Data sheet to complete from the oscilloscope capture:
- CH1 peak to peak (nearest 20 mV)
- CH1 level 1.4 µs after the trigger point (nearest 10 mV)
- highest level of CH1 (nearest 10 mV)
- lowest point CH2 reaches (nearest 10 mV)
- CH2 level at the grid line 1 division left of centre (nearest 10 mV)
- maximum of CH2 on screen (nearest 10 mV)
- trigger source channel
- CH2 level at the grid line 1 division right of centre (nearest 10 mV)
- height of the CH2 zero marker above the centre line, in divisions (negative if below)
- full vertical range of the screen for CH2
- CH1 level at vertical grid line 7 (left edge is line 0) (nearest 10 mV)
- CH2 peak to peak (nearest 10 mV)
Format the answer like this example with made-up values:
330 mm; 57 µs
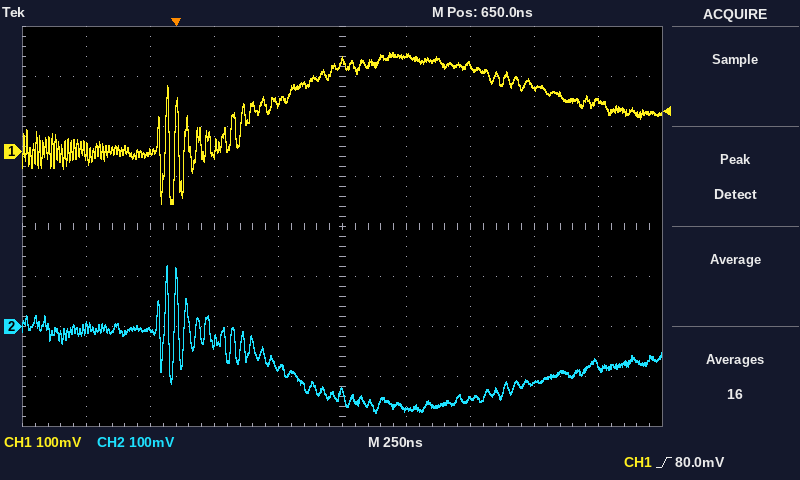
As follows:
300 mV; 130 mV; 200 mV; -170 mV; -80 mV; 120 mV; CH1; -170 mV; -2.0 div; 800 mV; 170 mV; 290 mV
